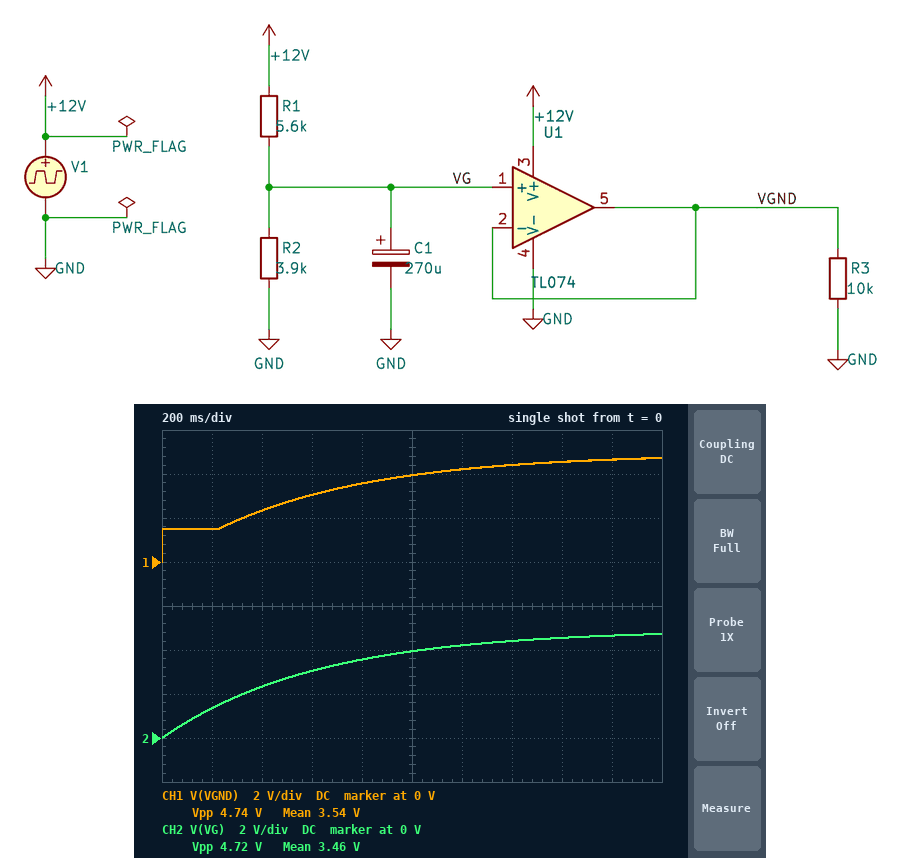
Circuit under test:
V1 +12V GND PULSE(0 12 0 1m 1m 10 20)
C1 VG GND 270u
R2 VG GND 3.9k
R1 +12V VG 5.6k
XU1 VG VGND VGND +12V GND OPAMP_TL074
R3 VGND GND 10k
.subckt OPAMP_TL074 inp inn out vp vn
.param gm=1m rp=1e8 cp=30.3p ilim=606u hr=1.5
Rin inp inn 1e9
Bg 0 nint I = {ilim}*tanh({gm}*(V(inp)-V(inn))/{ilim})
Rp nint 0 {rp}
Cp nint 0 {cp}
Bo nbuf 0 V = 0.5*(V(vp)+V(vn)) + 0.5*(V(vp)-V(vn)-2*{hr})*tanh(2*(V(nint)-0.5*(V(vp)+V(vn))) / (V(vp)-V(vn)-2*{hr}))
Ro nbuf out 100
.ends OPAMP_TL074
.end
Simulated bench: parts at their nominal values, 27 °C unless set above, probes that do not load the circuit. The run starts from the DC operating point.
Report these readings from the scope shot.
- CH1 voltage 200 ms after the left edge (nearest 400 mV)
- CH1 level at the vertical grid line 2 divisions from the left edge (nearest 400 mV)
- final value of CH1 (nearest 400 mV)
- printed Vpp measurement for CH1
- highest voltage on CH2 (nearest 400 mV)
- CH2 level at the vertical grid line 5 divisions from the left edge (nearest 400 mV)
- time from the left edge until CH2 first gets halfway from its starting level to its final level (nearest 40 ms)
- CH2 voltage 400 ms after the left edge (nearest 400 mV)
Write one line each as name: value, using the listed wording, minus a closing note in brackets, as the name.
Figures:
CH1 voltage 200 ms after the left edge: 1.6 V
CH1 level at the vertical grid line 2 divisions from the left edge: 2.4 V
final value of CH1: 4.8 V
printed Vpp measurement for CH1: 4.74 V
highest voltage on CH2: 4.8 V
CH2 level at the vertical grid line 5 divisions from the left edge: 4.0 V
time from the left edge until CH2 first gets halfway from its starting level to its final level: 400 ms
CH2 voltage 400 ms after the left edge: 2.4 V
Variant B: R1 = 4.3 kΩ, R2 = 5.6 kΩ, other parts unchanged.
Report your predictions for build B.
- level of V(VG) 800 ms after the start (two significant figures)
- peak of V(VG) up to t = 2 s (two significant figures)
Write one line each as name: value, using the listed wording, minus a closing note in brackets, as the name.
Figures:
level of V(VG) 800 ms after the start: 4.8 V
peak of V(VG) up to t = 2 s: 6.5 V
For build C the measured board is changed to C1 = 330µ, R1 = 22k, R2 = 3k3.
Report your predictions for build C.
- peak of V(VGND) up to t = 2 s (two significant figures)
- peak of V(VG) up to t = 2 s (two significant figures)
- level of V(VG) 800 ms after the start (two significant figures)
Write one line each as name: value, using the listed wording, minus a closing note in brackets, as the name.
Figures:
peak of V(VGND) up to t = 2 s: 1.5 V
peak of V(VG) up to t = 2 s: 1.4 V
level of V(VG) 800 ms after the start: 890 mV
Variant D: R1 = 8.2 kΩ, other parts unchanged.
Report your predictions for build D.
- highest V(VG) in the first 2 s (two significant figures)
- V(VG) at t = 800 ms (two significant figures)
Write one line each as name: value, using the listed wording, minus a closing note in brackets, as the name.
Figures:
highest V(VG) in the first 2 s: 3.6 V
V(VG) at t = 800 ms: 2.6 V
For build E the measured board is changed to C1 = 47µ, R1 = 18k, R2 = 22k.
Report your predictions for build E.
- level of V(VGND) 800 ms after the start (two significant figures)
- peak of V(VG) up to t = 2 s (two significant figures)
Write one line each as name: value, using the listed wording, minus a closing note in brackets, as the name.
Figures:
level of V(VGND) 800 ms after the start: 5.4 V
peak of V(VG) up to t = 2 s: 6.5 V
